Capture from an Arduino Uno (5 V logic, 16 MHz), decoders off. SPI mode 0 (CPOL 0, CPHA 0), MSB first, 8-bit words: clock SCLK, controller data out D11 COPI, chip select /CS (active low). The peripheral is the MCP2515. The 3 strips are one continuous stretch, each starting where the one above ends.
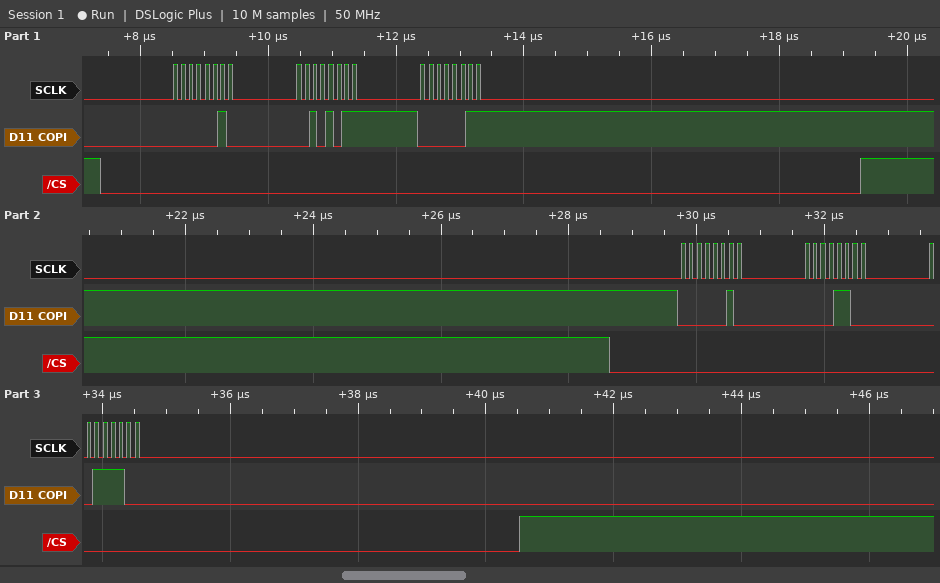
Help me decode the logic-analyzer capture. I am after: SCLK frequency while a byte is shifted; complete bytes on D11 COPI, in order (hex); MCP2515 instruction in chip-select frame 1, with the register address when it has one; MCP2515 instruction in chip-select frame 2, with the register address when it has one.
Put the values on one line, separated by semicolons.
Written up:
8 MHz; 02 2B 03 02 0C 3C; WRITE 0x2B; WRITE 0x0C
